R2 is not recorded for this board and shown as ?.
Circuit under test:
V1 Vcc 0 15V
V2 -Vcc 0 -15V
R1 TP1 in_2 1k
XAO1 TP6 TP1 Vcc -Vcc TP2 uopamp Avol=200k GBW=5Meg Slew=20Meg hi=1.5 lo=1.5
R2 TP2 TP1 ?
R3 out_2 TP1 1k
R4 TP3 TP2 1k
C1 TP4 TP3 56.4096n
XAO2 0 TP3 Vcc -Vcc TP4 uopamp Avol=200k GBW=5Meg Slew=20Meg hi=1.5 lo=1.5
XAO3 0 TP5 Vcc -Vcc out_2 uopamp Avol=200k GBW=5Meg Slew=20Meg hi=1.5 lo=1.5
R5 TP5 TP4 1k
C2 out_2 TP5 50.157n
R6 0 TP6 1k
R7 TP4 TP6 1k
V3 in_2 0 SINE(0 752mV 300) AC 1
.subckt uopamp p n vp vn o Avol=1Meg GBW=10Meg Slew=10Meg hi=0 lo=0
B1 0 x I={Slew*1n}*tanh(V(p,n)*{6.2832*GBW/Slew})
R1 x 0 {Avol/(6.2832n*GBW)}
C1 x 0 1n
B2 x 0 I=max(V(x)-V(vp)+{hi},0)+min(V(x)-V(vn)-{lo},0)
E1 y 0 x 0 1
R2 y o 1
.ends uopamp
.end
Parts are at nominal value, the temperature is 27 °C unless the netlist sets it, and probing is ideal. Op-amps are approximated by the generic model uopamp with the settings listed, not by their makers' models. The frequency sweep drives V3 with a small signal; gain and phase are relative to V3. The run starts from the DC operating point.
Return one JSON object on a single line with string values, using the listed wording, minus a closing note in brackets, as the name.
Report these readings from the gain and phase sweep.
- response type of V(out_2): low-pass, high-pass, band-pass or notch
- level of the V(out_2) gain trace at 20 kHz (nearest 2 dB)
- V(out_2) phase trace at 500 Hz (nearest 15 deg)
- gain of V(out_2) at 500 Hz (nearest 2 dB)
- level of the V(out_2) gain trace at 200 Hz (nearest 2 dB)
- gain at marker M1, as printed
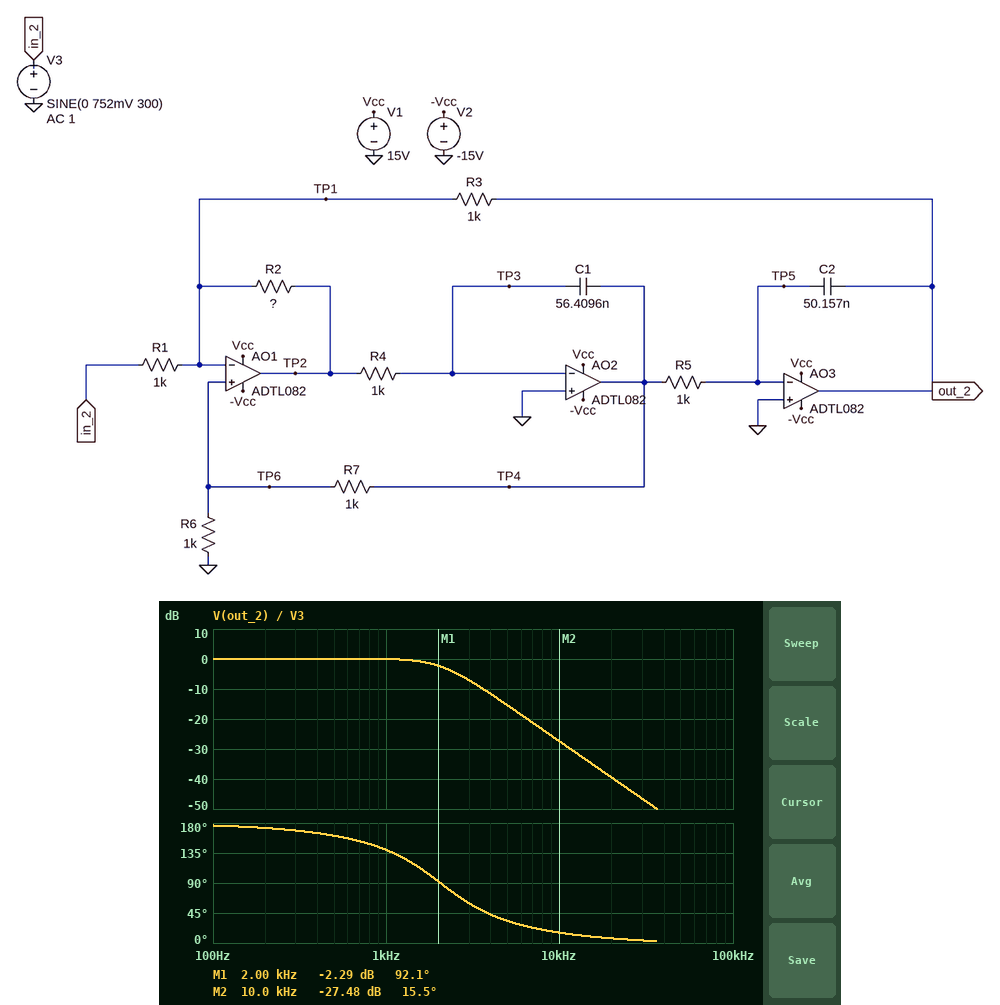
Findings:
{"response type of V(out_2): low-pass, high-pass, band-pass or notch": "low-pass", "level of the V(out_2) gain trace at 20 kHz": "-40 dB", "V(out_2) phase trace at 500 Hz": "165 deg", "gain of V(out_2) at 500 Hz": "0 dB", "level of the V(out_2) gain trace at 200 Hz": "0 dB", "gain at marker M1, as printed": "-2.29 dB"}
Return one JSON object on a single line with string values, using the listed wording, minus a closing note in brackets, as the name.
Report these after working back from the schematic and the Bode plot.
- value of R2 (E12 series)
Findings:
{"value of R2": "470 Ω"}
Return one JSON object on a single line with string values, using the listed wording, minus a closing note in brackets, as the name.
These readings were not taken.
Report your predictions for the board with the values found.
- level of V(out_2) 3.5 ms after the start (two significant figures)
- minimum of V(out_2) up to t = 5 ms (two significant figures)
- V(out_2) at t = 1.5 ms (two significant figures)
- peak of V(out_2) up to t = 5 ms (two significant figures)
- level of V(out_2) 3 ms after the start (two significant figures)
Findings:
{"level of V(out_2) 3.5 ms after the start": "-88 mV", "minimum of V(out_2) up to t = 5 ms": "-750 mV", "V(out_2) at t = 1.5 ms": "-370 mV", "peak of V(out_2) up to t = 5 ms": "750 mV", "level of V(out_2) 3 ms after the start": "550 mV"}
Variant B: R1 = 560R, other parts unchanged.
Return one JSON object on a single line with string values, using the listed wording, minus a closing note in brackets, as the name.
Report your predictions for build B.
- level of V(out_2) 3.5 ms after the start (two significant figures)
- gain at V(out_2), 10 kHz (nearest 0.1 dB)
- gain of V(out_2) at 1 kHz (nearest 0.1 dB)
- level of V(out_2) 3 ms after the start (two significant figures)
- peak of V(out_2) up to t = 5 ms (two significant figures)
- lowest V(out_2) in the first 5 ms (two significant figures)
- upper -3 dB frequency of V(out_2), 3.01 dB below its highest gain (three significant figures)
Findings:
{"level of V(out_2) 3.5 ms after the start": "-110 mV", "gain at V(out_2), 10 kHz": "-22.6 dB", "gain of V(out_2) at 1 kHz": "4.3 dB", "level of V(out_2) 3 ms after the start": "1.0 V", "peak of V(out_2) up to t = 5 ms": "1.3 V", "lowest V(out_2) in the first 5 ms": "-1.3 V", "upper -3 dB frequency of V(out_2), 3.01 dB below its highest gain": "1.80 kHz"}
